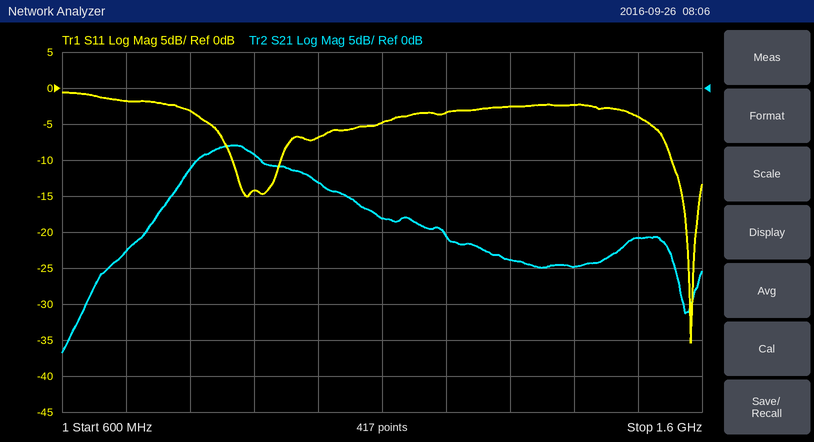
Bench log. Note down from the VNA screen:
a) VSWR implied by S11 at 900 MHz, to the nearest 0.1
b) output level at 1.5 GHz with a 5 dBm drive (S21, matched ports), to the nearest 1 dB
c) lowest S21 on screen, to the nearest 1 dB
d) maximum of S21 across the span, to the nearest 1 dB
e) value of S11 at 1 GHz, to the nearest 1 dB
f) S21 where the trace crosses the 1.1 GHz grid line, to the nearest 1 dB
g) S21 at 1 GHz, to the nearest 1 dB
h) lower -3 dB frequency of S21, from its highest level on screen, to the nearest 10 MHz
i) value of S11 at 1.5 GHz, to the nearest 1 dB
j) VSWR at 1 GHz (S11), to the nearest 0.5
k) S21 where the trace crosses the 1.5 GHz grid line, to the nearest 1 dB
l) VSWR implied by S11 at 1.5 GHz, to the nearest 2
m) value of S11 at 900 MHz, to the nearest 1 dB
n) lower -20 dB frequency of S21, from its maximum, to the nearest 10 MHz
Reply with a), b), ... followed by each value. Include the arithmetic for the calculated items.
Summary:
a) |Γ| = 10^(-14/20) = 0.1995; VSWR = (1 + 0.1995)/(1 − 0.1995) ≈ 1.5
b) 5 dBm + (-21 dB) = -16 dBm
c) -37 dB
d) -8 dB
e) -7 dB
f) -18 dB
g) -13 dB
h) 800 MHz
i) -4 dB
j) |Γ| = 10^(-7/20) = 0.4467; VSWR = (1 + 0.4467)/(1 − 0.4467) ≈ 2.61, so 2.5 to the nearest 0.5
k) -21 dB
l) |Γ| = 10^(-4/20) = 0.6310; VSWR = (1 + 0.6310)/(1 − 0.6310) ≈ 4
m) -14 dB
n) 650 MHz
